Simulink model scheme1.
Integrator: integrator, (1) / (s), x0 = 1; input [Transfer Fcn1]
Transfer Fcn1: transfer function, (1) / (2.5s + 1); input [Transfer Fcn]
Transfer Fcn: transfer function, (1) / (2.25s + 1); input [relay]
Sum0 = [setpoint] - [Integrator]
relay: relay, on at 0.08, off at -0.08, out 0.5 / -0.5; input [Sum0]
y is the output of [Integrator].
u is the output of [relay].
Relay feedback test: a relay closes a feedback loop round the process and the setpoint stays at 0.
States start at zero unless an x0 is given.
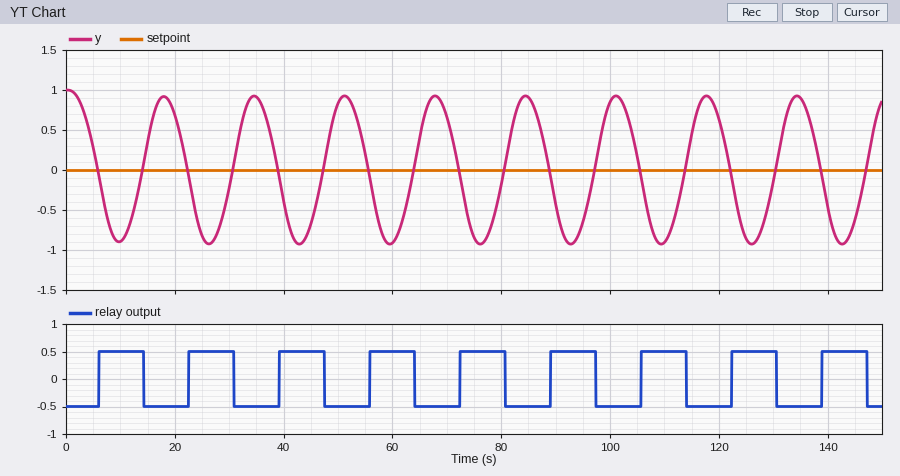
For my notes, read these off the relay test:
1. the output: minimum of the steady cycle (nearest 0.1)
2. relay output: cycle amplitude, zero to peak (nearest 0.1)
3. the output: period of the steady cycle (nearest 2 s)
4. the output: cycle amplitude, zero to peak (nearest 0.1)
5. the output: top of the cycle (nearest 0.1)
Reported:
-0.9
0.5
16 s
0.9
0.9
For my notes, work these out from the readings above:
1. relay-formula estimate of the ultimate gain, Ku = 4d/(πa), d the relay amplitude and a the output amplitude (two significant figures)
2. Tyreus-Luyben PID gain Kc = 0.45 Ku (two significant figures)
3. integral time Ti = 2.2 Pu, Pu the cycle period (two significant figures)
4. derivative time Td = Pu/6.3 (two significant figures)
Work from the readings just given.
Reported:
0.71
0.32
35 s
2.5 s
